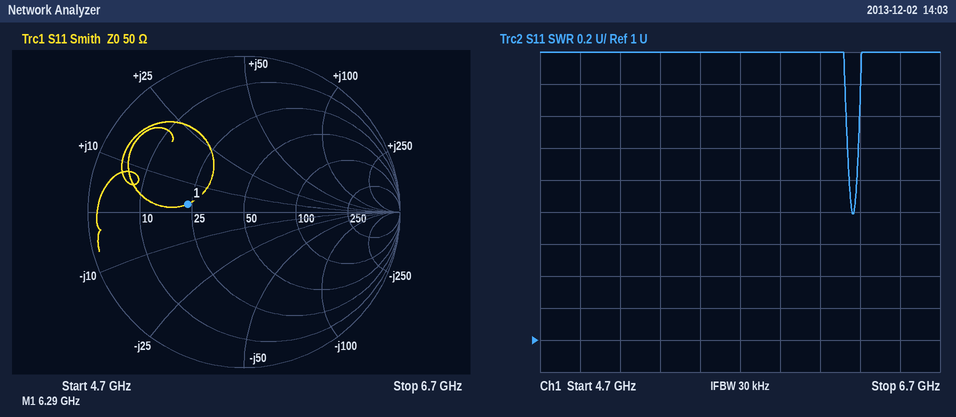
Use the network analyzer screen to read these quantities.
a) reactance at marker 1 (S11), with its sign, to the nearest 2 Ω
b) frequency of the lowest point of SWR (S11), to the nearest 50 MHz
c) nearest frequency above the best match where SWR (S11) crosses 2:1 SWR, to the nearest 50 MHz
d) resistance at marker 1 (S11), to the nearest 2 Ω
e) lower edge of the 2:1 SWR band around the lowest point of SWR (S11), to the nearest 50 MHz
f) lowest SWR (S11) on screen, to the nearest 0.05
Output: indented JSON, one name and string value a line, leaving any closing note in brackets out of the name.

{
  "reactance at marker 1 (S11), with its sign, to the nearest 2 Ω": "+2 Ω",
  "frequency of the lowest point of SWR (S11), to the nearest 50 MHz": "6.25 GHz",
  "nearest frequency above the best match where SWR (S11) crosses 2:1 SWR, to the nearest 50 MHz": "6.30 GHz",
  "resistance at marker 1 (S11), to the nearest 2 Ω": "24 Ω",
  "lower edge of the 2:1 SWR band around the lowest point of SWR (S11), to the nearest 50 MHz": "6.25 GHz",
  "lowest SWR (S11) on screen, to the nearest 0.05": "1.80"
}
